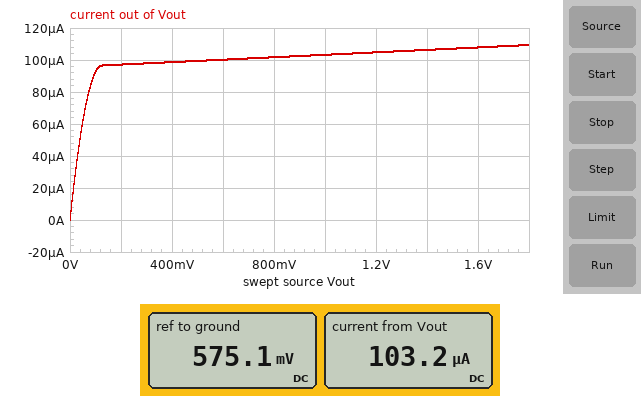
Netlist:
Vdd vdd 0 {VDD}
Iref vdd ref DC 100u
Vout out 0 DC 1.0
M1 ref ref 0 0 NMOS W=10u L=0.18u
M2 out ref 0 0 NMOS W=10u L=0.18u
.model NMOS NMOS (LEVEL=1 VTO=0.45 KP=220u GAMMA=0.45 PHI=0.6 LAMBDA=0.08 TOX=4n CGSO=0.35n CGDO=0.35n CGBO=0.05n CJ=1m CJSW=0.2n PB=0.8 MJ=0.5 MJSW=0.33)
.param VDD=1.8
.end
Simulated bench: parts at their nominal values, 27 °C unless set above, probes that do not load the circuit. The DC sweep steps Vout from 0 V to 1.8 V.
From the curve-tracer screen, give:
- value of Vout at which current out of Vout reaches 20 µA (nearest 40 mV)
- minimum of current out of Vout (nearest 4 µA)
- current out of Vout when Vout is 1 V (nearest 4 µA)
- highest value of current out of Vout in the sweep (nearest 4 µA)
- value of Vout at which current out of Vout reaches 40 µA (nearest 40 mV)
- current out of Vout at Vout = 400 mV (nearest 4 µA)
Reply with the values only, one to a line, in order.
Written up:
0 V
0 A
104 µA
108 µA
40 mV
100 µA
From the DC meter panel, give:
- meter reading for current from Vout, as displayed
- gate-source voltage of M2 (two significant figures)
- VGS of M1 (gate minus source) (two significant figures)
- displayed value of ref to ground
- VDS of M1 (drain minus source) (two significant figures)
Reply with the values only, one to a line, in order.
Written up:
103.2 µA
580 mV
580 mV
575.1 mV
580 mV
